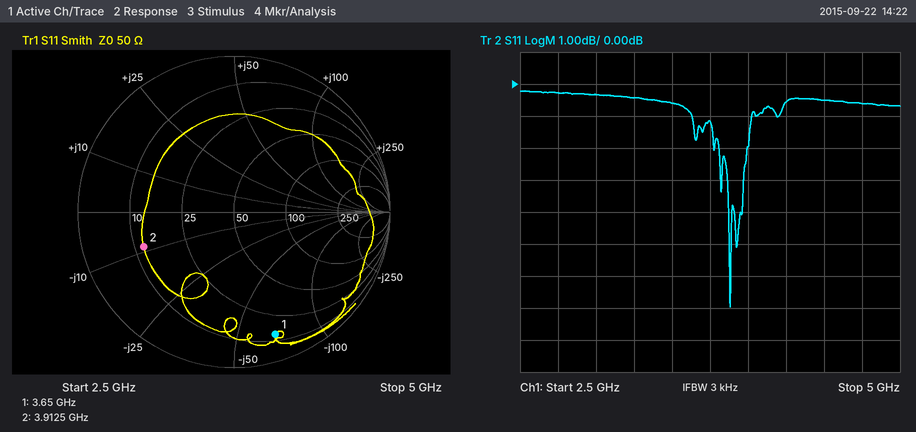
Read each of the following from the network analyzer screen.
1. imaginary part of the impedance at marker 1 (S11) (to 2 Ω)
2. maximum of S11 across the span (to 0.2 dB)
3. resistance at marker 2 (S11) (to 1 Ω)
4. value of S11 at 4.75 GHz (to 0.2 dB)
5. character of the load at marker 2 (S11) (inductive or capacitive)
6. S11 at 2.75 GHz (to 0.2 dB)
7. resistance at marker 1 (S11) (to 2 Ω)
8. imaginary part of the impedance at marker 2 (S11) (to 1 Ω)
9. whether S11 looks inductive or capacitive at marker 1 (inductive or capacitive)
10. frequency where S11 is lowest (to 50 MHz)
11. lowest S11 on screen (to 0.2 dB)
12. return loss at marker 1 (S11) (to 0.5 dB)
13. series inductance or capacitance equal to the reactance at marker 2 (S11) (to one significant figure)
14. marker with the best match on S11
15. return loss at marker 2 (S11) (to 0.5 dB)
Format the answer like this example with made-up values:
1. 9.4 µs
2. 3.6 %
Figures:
1. -68 Ω
2. -0.2 dB
3. 12 Ω
4. -0.6 dB
5. capacitive
6. -0.2 dB
7. 14 Ω
8. -9 Ω
9. capacitive
10. 3.90 GHz
11. -7.0 dB
12. 1.5 dB
13. 5 pF
14. marker 2
15. 4.0 dB
